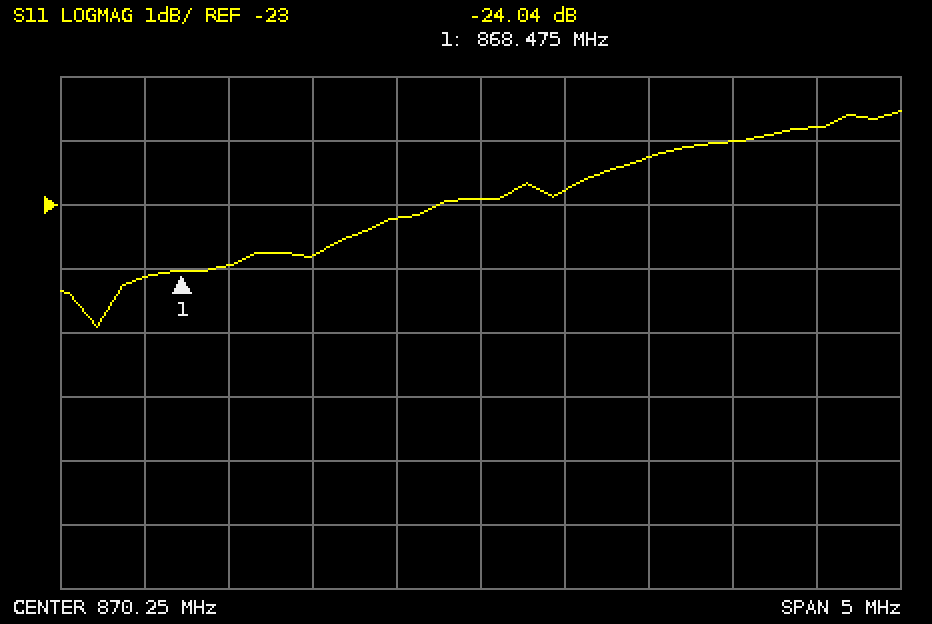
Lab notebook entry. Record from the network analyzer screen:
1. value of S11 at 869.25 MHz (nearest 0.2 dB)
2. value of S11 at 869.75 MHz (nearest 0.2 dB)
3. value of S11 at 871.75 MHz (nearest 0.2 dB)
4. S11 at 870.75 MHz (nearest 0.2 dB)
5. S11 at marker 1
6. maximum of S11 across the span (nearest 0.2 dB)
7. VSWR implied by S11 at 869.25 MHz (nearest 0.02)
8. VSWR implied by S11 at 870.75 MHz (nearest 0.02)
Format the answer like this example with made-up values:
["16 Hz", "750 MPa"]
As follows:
["-23.8 dB", "-23.2 dB", "-22.0 dB", "-22.8 dB", "-24.04 dB", "-21.6 dB", "1.14", "1.16"]
